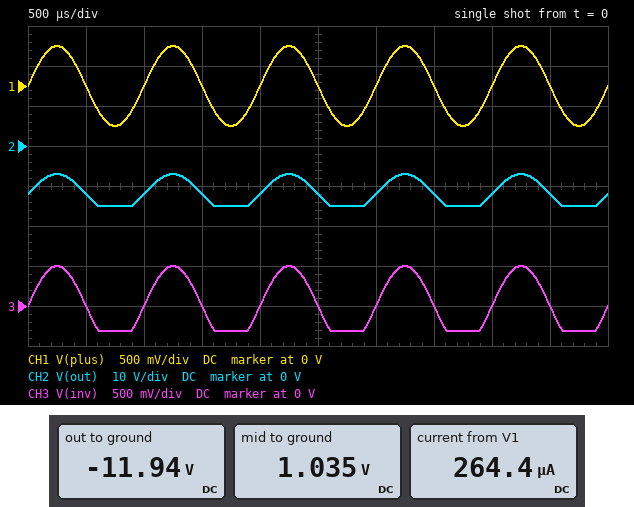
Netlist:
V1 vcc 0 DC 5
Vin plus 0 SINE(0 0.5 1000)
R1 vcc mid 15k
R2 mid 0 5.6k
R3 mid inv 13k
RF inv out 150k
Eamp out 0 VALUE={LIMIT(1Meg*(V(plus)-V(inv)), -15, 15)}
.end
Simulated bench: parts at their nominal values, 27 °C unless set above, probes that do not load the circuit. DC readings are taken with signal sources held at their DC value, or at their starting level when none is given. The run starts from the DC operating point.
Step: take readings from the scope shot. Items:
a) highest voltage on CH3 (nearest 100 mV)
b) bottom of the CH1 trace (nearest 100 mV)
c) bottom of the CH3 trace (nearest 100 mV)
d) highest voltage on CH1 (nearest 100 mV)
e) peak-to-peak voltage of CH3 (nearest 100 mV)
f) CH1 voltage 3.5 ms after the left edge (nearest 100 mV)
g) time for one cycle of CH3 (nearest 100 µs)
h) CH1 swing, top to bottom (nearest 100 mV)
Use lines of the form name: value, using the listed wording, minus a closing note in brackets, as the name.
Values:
highest voltage on CH3: 500 mV
bottom of the CH1 trace: -500 mV
bottom of the CH3 trace: -300 mV
highest voltage on CH1: 500 mV
peak-to-peak voltage of CH3: 800 mV
CH1 voltage 3.5 ms after the left edge: 0 V
time for one cycle of CH3: 1.0 ms
CH1 swing, top to bottom: 1.0 V
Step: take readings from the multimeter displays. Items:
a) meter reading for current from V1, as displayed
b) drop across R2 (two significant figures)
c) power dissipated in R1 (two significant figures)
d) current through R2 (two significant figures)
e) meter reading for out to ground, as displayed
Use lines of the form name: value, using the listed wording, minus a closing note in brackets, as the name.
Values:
meter reading for current from V1, as displayed: 264.4 µA
drop across R2: 1.0 V
power dissipated in R1: 1.0 mW
current through R2: 180 µA
meter reading for out to ground, as displayed: -11.94 V
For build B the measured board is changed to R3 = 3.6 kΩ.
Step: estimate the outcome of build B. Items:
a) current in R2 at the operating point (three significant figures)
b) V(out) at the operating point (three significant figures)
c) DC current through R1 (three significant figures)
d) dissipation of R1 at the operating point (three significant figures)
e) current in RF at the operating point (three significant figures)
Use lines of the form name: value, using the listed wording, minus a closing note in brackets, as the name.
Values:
current in R2 at the operating point: 167 µA
V(out) at the operating point: -15.0 V
DC current through R1: 271 µA
dissipation of R1 at the operating point: 1.10 mW
current in RF at the operating point: 104 µA
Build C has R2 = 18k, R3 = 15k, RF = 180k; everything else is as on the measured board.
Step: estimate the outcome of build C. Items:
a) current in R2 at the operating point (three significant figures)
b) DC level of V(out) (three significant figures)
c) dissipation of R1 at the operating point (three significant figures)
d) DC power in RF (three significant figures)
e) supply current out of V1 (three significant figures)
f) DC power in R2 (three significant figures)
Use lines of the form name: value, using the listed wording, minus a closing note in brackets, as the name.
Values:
current in R2 at the operating point: 112 µA
DC level of V(out): -15.0 V
dissipation of R1 at the operating point: 595 µW
DC power in RF: 1.37 mW
supply current out of V1: 199 µA
DC power in R2: 225 µW
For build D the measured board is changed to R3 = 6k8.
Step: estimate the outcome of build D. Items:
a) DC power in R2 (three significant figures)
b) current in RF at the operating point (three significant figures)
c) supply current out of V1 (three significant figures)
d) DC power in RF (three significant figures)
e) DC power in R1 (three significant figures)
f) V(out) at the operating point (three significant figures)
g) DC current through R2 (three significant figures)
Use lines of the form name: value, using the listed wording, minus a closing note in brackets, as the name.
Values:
DC power in R2: 159 µW
current in RF at the operating point: 102 µA
supply current out of V1: 270 µA
DC power in RF: 1.55 mW
DC power in R1: 1.10 mW
V(out) at the operating point: -15.0 V
DC current through R2: 169 µA
